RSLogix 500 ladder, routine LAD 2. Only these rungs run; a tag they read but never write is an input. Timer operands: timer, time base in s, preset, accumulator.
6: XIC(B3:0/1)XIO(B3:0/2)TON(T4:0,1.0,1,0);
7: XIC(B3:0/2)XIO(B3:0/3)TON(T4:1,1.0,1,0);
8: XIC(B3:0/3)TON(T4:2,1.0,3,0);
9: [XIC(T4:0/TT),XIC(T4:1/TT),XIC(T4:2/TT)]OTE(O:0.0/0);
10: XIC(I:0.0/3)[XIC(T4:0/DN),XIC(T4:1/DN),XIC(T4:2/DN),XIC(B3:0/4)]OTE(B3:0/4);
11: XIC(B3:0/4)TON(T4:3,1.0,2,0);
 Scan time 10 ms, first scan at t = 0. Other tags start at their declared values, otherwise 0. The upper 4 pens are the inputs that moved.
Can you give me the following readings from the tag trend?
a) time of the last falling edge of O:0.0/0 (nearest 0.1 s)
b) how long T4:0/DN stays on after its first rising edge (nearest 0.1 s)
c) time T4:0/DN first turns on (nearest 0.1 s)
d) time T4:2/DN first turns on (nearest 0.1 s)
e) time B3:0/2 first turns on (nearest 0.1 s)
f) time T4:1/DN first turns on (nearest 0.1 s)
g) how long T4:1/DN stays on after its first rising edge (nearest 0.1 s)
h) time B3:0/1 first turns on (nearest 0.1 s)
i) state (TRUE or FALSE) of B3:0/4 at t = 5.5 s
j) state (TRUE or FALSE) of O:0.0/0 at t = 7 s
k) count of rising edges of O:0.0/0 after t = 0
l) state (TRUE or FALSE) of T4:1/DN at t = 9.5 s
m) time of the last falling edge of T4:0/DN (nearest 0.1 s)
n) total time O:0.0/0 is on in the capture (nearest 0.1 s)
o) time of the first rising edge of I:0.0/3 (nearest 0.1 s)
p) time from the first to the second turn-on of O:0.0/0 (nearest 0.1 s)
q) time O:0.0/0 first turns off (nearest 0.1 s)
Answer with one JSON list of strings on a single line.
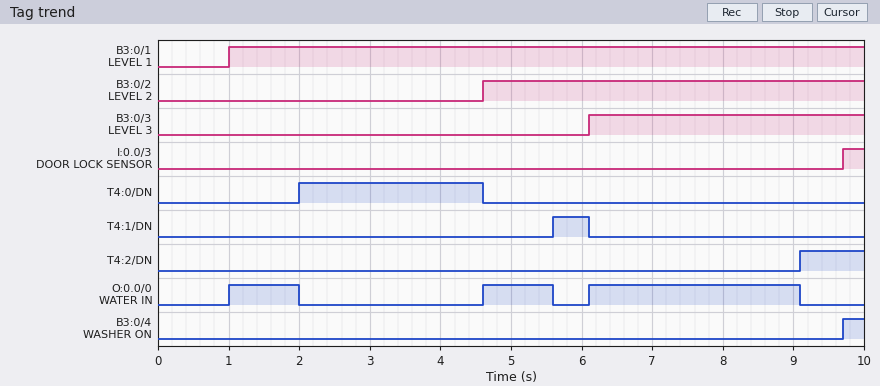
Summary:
["9.1 s", "2.6 s", "2.0 s", "9.1 s", "4.6 s", "5.6 s", "0.5 s", "1.0 s", "FALSE", "TRUE", "3", "FALSE", "4.6 s", "5.0 s", "9.7 s", "3.6 s", "2.0 s"]
